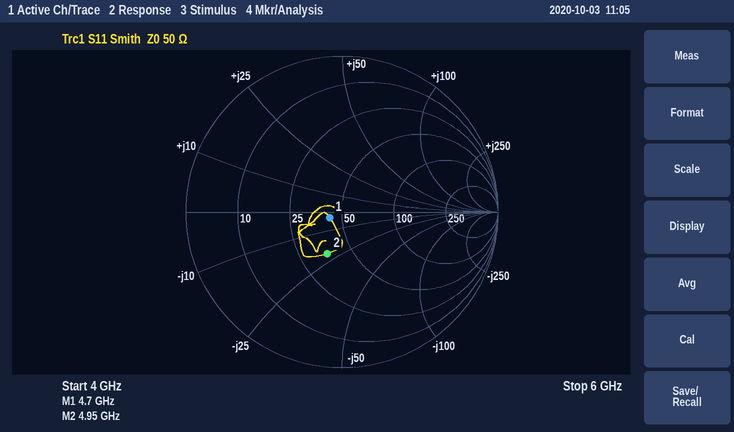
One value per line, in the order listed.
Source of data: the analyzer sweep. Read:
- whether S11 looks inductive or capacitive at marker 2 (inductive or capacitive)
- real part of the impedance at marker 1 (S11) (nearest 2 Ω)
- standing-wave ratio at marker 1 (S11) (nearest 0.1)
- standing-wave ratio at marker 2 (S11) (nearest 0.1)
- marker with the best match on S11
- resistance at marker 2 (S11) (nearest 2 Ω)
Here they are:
capacitive
42 Ω
1.2
1.8
marker 1
36 Ω
